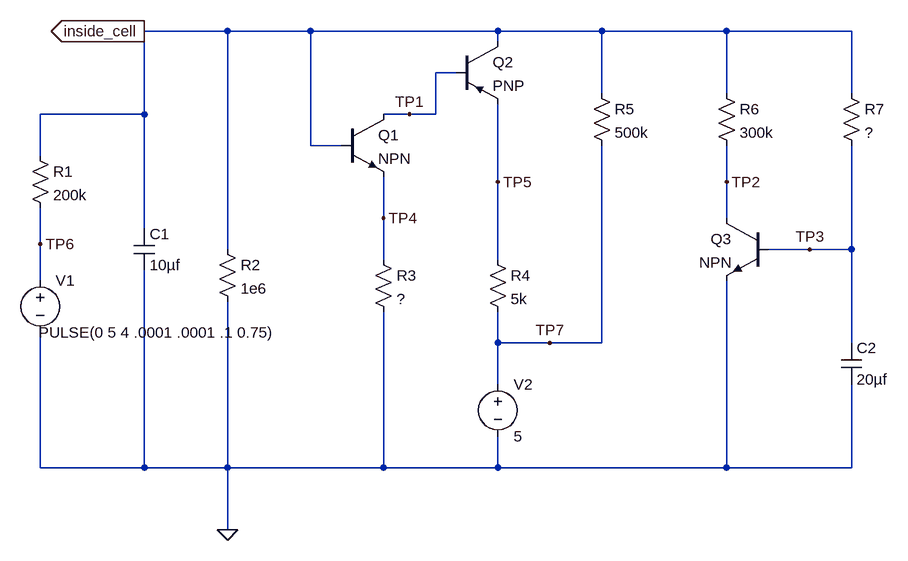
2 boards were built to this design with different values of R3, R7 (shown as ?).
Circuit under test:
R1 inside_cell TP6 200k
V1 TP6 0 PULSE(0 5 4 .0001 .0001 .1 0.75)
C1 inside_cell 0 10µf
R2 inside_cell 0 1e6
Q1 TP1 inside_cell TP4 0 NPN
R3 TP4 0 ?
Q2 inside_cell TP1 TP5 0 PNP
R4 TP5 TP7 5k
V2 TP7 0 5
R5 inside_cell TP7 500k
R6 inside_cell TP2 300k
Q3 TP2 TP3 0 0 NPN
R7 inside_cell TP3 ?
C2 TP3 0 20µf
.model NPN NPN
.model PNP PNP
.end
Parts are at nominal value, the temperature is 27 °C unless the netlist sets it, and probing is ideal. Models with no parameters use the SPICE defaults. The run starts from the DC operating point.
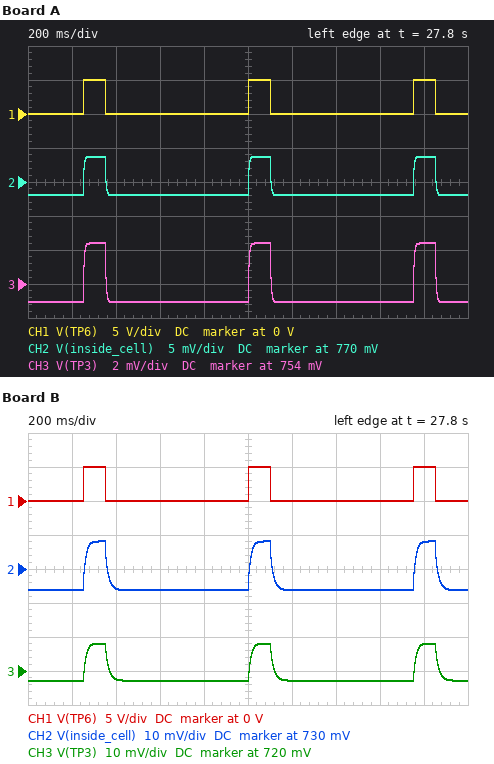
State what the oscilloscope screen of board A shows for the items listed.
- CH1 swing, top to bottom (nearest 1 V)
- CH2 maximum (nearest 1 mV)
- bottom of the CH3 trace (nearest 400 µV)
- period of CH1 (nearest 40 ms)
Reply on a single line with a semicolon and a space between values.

5 V; 774 mV; 752.8 mV; 760 ms
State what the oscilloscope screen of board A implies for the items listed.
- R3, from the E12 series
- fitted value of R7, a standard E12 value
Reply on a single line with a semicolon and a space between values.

68 kΩ; 68 Ω
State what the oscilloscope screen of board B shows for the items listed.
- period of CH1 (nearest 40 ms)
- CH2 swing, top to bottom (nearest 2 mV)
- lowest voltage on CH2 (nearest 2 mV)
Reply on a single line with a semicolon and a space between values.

760 ms; 14 mV; 724 mV
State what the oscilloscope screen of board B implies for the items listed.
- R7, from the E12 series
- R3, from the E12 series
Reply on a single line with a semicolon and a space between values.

120 Ω; 270 kΩ
